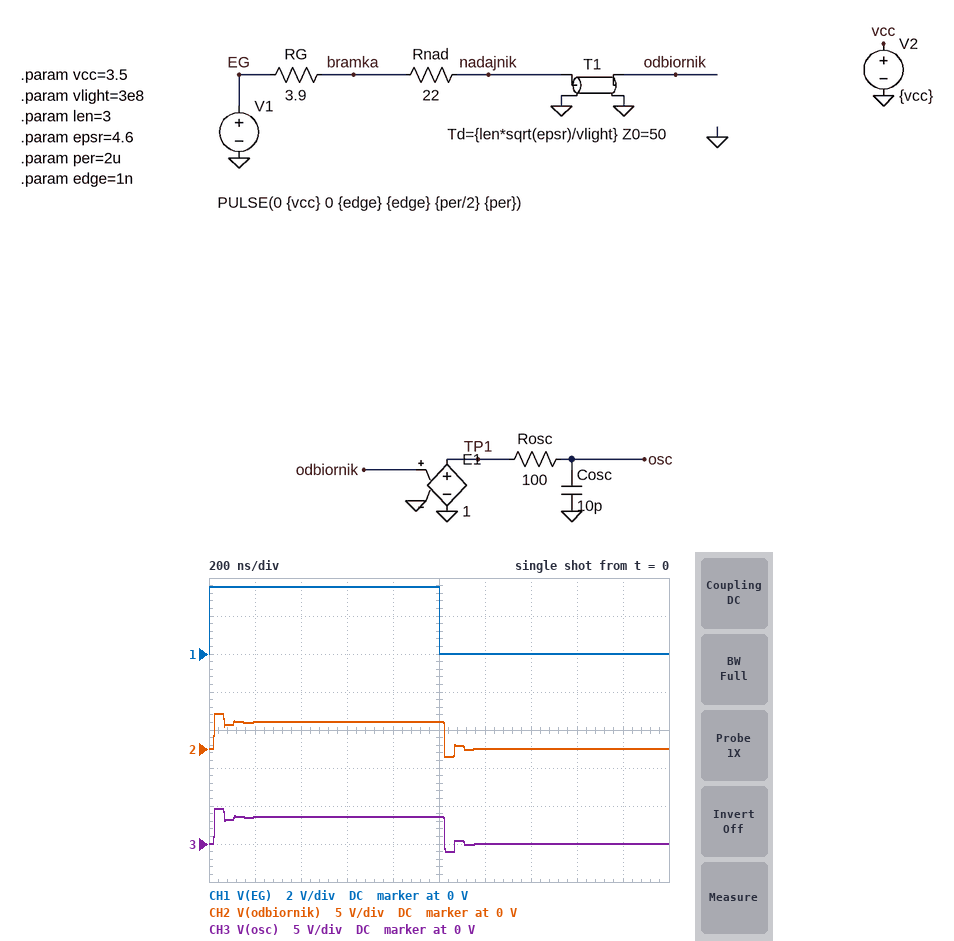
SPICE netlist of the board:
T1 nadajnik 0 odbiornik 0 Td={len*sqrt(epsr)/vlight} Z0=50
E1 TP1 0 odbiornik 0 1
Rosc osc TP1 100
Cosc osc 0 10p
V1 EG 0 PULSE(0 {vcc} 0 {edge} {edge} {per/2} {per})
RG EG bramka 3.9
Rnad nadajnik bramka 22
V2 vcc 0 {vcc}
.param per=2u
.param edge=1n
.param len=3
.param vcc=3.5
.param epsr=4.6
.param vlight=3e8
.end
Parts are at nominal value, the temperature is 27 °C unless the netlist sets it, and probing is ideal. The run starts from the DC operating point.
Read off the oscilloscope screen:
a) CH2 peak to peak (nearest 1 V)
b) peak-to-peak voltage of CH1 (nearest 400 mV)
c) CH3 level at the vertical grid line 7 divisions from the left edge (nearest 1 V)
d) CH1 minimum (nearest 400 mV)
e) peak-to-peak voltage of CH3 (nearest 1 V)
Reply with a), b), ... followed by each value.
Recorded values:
a) 6 V
b) 3.6 V
c) 0 V
d) 0 V
e) 6 V
